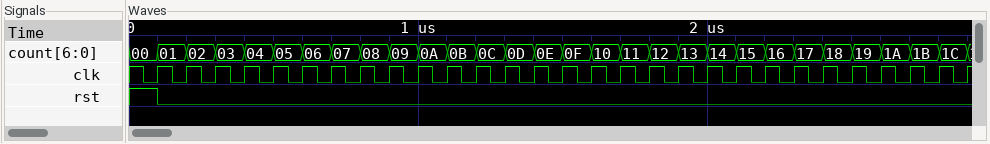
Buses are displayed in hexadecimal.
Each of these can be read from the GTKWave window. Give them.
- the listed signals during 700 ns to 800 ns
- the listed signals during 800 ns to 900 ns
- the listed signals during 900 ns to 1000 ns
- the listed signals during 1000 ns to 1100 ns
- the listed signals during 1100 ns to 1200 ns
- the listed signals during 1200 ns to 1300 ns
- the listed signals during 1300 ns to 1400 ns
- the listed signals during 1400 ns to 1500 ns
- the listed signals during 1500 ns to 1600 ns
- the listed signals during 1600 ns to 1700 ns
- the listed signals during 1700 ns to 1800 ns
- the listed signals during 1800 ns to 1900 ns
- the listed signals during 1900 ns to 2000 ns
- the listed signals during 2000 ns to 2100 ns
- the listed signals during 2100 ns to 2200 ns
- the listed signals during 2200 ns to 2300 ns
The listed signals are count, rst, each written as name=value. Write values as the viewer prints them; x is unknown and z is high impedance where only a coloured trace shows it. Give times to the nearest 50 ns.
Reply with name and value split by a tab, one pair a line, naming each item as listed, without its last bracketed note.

the listed signals during 700 ns to 800 ns	count=07, rst=0
the listed signals during 800 ns to 900 ns	count=08, rst=0
the listed signals during 900 ns to 1000 ns	count=09, rst=0
the listed signals during 1000 ns to 1100 ns	count=0A, rst=0
the listed signals during 1100 ns to 1200 ns	count=0B, rst=0
the listed signals during 1200 ns to 1300 ns	count=0C, rst=0
the listed signals during 1300 ns to 1400 ns	count=0D, rst=0
the listed signals during 1400 ns to 1500 ns	count=0E, rst=0
the listed signals during 1500 ns to 1600 ns	count=0F, rst=0
the listed signals during 1600 ns to 1700 ns	count=10, rst=0
the listed signals during 1700 ns to 1800 ns	count=11, rst=0
the listed signals during 1800 ns to 1900 ns	count=12, rst=0
the listed signals during 1900 ns to 2000 ns	count=13, rst=0
the listed signals during 2000 ns to 2100 ns	count=14, rst=0
the listed signals during 2100 ns to 2200 ns	count=15, rst=0
the listed signals during 2200 ns to 2300 ns	count=16, rst=0
